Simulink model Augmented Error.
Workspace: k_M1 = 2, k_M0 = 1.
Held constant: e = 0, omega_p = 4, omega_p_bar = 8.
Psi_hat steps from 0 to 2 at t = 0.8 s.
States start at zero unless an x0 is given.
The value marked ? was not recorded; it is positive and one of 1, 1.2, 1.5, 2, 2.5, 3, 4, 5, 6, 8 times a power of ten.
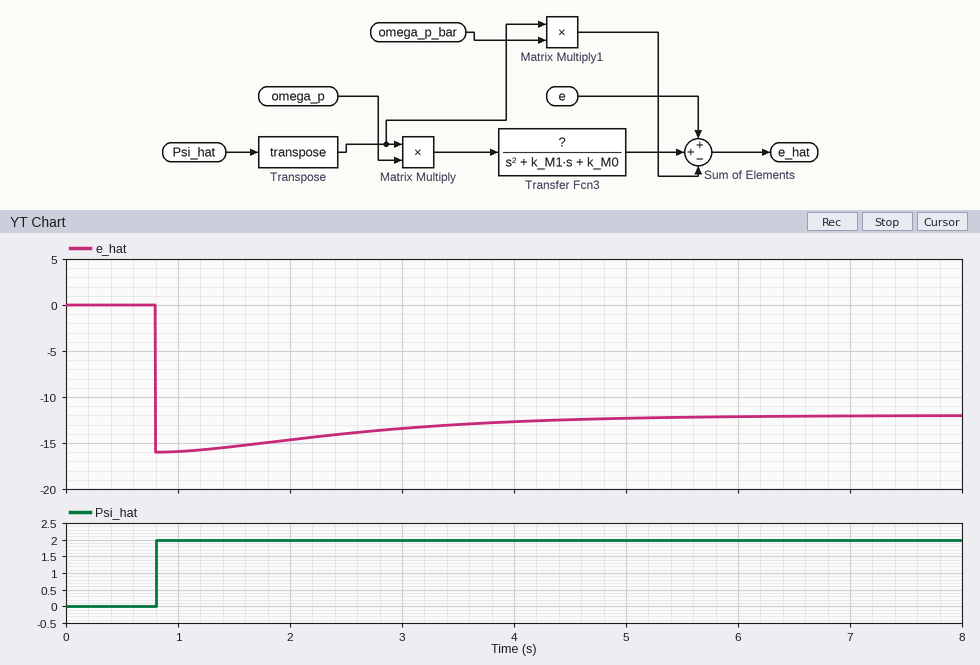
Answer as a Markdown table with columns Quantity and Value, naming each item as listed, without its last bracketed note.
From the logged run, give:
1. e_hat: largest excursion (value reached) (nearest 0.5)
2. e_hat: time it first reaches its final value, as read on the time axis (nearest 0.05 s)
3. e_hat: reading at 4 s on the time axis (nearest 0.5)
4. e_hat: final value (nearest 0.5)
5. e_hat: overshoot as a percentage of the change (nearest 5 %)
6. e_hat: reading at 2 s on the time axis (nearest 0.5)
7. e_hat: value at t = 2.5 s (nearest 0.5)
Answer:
| Quantity | Value |
|---|---|
| e_hat: largest excursion (value reached) | -16.0 |
| e_hat: time it first reaches its final value, as read on the time axis | 0.80 s |
| e_hat: reading at 4 s on the time axis | -12.5 |
| e_hat: final value | -12.0 |
| e_hat: overshoot as a percentage of the change | 35 % |
| e_hat: reading at 2 s on the time axis | -14.5 |
| e_hat: value at t = 2.5 s | -14.0 |
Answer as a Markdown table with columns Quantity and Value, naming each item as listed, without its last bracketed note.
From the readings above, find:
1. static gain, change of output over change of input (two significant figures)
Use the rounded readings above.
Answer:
| Quantity | Value |
|---|---|
| static gain, change of output over change of input | -6.0 |
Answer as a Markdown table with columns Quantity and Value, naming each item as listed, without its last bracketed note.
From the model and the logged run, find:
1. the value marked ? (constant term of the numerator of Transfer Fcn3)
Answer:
| Quantity | Value |
|---|---|
| the value marked ? | 0.5 |
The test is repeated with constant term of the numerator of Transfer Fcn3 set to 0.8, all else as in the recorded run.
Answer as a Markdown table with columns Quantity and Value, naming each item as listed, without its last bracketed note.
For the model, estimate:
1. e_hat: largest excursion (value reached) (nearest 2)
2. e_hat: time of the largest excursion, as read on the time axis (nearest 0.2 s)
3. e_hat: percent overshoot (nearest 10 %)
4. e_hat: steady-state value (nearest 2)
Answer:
| Quantity | Value |
|---|---|
| e_hat: largest excursion (value reached) | -16 |
| e_hat: time of the largest excursion, as read on the time axis | 0.8 s |
| e_hat: percent overshoot | 70 % |
| e_hat: steady-state value | -10 |
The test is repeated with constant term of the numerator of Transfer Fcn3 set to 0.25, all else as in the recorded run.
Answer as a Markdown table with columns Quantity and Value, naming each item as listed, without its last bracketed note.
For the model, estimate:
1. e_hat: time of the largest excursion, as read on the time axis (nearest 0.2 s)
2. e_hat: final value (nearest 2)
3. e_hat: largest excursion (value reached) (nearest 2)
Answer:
| Quantity | Value |
|---|---|
| e_hat: time of the largest excursion, as read on the time axis | 0.8 s |
| e_hat: final value | -14 |
| e_hat: largest excursion (value reached) | -16 |
